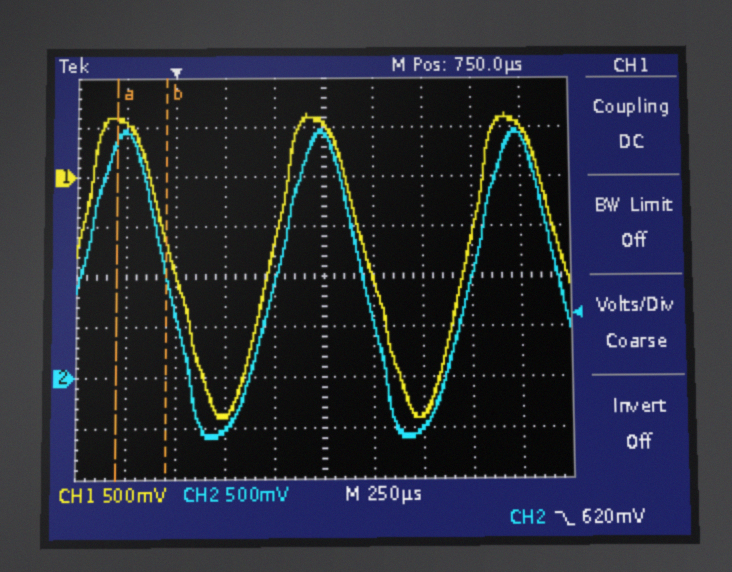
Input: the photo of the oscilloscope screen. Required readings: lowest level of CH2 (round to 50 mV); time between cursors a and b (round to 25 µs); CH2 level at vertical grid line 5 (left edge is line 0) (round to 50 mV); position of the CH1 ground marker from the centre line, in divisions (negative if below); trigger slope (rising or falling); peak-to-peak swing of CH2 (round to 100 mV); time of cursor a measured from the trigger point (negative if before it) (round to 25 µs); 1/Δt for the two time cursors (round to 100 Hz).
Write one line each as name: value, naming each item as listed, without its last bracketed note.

lowest level of CH2: -600 mV
time between cursors a and b: 250 µs
CH2 level at vertical grid line 5 (left edge is line 0): 2.45 V
position of the CH1 ground marker from the centre line, in divisions: +2.0 div
trigger slope: falling
peak-to-peak swing of CH2: 3.10 V
time of cursor a measured from the trigger point (negative if before it): -300 µs
1/Δt for the two time cursors: 4.0 kHz
